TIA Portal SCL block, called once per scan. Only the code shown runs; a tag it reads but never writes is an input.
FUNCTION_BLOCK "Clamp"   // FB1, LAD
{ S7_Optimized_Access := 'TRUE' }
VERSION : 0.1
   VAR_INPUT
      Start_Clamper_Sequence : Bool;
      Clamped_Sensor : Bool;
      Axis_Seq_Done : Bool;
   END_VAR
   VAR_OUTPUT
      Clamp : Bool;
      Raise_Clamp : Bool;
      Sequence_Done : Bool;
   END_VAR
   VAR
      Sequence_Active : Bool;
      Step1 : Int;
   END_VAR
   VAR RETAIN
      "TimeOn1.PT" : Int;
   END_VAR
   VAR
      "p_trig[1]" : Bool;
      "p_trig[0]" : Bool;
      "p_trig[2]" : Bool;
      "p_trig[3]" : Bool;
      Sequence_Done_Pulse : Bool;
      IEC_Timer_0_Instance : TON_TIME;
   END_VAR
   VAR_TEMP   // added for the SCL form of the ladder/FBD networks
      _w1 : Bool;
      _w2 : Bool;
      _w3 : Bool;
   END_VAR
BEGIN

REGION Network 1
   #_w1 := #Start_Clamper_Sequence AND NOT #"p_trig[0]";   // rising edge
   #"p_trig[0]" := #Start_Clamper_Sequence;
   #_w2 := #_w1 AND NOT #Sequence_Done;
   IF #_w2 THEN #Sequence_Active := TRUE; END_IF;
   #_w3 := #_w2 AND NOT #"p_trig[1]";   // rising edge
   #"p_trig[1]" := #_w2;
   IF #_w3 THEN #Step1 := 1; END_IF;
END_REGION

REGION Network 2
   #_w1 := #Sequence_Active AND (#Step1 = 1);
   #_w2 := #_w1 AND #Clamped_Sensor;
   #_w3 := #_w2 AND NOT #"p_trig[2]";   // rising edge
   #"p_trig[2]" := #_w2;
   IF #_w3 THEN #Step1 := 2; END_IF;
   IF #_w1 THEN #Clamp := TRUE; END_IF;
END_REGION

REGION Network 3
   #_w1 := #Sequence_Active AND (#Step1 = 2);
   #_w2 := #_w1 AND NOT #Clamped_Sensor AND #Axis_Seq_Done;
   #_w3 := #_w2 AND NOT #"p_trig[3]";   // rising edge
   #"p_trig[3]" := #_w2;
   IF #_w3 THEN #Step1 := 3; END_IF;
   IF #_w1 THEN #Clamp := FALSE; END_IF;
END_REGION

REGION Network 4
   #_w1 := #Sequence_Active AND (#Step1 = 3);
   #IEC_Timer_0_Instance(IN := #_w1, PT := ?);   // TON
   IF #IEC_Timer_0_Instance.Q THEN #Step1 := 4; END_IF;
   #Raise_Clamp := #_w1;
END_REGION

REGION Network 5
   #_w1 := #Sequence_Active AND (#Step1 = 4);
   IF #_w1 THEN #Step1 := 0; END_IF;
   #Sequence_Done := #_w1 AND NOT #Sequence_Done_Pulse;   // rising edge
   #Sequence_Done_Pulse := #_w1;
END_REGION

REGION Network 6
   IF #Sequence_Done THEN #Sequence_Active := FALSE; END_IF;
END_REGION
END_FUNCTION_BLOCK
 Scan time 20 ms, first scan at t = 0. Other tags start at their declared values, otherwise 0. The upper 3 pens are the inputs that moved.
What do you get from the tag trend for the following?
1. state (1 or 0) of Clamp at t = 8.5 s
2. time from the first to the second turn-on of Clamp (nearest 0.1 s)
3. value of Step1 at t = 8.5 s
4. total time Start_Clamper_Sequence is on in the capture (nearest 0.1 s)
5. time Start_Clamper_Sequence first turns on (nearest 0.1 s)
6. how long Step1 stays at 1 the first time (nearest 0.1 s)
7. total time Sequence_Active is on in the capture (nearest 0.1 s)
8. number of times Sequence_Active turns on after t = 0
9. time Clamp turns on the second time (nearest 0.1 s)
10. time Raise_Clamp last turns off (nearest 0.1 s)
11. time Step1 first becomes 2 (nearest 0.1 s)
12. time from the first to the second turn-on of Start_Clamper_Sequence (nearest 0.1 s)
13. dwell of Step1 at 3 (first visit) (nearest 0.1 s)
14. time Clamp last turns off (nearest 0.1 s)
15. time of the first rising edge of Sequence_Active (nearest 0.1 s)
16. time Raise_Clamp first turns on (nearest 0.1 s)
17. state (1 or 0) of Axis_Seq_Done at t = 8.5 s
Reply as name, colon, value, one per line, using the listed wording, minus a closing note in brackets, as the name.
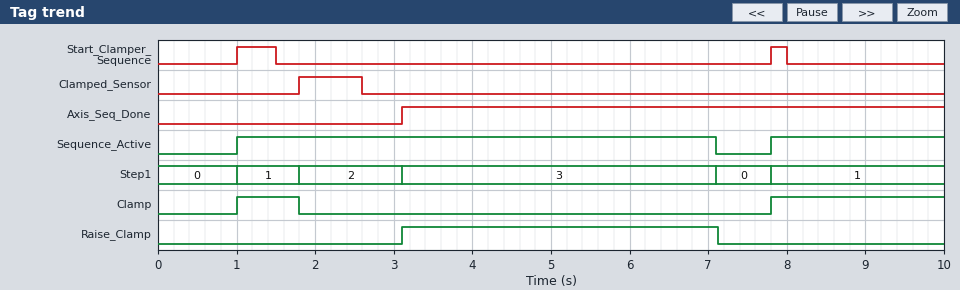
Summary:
state (1 or 0) of Clamp at t = 8.5 s: 1
time from the first to the second turn-on of Clamp: 6.8 s
value of Step1 at t = 8.5 s: 1
total time Start_Clamper_Sequence is on in the capture: 0.7 s
time Start_Clamper_Sequence first turns on: 1.0 s
how long Step1 stays at 1 the first time: 0.8 s
total time Sequence_Active is on in the capture: 8.3 s
number of times Sequence_Active turns on after t = 0: 2
time Clamp turns on the second time: 7.8 s
time Raise_Clamp last turns off: 7.1 s
time Step1 first becomes 2: 1.8 s
time from the first to the second turn-on of Start_Clamper_Sequence: 6.8 s
dwell of Step1 at 3 (first visit): 4.0 s
time Clamp last turns off: 1.8 s
time of the first rising edge of Sequence_Active: 1.0 s
time Raise_Clamp first turns on: 3.1 s
state (1 or 0) of Axis_Seq_Done at t = 8.5 s: 1
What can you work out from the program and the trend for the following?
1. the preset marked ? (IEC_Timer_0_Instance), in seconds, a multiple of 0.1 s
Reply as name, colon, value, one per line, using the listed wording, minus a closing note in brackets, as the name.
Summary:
the preset marked ? (IEC_Timer_0_Instance), in seconds, a multiple of 0.1 s: 4.0 s
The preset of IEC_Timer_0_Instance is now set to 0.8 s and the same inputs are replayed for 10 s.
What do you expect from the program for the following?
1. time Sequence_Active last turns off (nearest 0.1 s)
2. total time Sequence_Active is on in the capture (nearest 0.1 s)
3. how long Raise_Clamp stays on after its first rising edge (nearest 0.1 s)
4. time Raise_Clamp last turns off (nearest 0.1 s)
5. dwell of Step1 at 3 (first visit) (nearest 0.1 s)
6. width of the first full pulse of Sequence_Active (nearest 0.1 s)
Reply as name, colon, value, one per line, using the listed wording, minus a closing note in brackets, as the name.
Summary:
time Sequence_Active last turns off: 3.9 s
total time Sequence_Active is on in the capture: 5.1 s
how long Raise_Clamp stays on after its first rising edge: 0.8 s
time Raise_Clamp last turns off: 3.9 s
dwell of Step1 at 3 (first visit): 0.8 s
width of the first full pulse of Sequence_Active: 2.9 s
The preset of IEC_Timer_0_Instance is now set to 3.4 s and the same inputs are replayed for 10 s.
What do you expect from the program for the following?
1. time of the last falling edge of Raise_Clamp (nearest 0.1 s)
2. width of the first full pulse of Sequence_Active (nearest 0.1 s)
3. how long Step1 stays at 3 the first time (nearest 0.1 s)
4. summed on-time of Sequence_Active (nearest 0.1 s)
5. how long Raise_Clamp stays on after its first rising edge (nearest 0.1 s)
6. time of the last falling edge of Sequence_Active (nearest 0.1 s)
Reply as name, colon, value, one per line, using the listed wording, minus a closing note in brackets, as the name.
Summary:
time of the last falling edge of Raise_Clamp: 6.5 s
width of the first full pulse of Sequence_Active: 5.5 s
how long Step1 stays at 3 the first time: 3.4 s
summed on-time of Sequence_Active: 7.7 s
how long Raise_Clamp stays on after its first rising edge: 3.4 s
time of the last falling edge of Sequence_Active: 6.5 s
